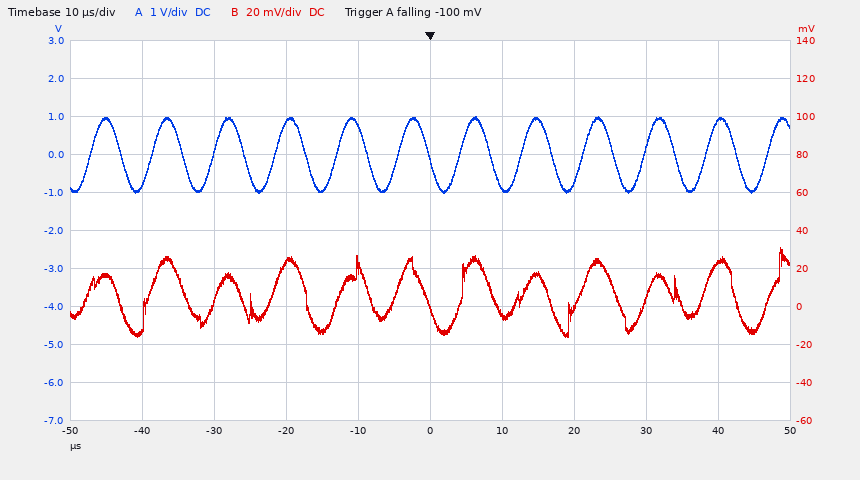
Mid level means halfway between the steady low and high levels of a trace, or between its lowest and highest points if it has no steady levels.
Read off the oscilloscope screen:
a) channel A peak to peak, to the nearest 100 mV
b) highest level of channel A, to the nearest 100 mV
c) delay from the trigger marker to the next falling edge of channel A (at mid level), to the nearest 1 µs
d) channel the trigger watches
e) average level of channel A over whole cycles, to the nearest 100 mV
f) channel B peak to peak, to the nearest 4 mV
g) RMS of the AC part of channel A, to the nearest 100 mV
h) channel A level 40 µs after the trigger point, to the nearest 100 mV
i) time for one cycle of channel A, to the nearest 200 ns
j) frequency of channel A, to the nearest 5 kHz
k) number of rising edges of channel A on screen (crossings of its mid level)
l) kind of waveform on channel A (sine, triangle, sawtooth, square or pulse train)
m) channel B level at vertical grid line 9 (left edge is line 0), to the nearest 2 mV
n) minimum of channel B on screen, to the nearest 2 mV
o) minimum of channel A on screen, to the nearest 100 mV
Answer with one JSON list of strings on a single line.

["2.0 V", "1.0 V", "8 µs", "channel A", "0.0 V", "48 mV", "700 mV", "900 mV", "8.6 µs", "115 kHz", "12", "sine", "24 mV", "-16 mV", "-1.0 V"]
